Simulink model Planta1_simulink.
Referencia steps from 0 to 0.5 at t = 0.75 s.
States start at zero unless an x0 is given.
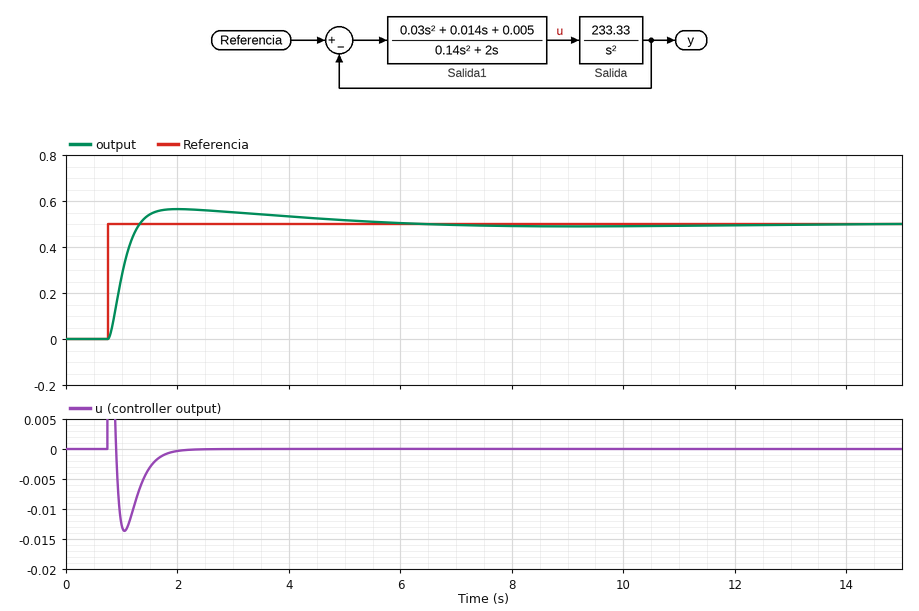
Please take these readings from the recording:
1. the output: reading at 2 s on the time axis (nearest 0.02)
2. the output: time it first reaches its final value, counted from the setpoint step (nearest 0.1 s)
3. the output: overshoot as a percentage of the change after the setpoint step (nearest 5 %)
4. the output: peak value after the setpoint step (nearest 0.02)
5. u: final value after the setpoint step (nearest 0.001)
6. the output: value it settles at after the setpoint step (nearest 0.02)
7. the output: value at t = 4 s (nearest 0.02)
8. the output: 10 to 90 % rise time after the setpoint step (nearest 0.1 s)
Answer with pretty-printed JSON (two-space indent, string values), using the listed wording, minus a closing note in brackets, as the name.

{
  "the output: reading at 2 s on the time axis": "0.56",
  "the output: time it first reaches its final value, counted from the setpoint step": "0.6 s",
  "the output: overshoot as a percentage of the change after the setpoint step": "15 %",
  "the output: peak value after the setpoint step": "0.56",
  "u: final value after the setpoint step": "0.000",
  "the output: value it settles at after the setpoint step": "0.50",
  "the output: value at t = 4 s": "0.54",
  "the output: 10 to 90 % rise time after the setpoint step": "0.4 s"
}
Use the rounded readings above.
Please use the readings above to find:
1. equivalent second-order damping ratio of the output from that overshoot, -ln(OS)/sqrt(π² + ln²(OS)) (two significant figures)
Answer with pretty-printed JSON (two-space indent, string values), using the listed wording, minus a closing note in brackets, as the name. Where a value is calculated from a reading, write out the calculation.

{
  "equivalent second-order damping ratio of the output from that overshoot, -ln(OS)/sqrt(π² + ln²(OS))": "ln(0.15) = -1.897; 1.897 / sqrt(9.870 + 3.599) = 0.52"
}
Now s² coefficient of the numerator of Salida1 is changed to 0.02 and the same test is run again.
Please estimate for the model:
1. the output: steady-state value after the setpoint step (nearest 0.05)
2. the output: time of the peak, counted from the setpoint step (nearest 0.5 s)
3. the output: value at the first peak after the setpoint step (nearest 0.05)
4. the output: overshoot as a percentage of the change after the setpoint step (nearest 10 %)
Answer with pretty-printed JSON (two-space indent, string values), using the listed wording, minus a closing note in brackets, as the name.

{
  "the output: steady-state value after the setpoint step": "0.50",
  "the output: time of the peak, counted from the setpoint step": "1.5 s",
  "the output: value at the first peak after the setpoint step": "0.60",
  "the output: overshoot as a percentage of the change after the setpoint step": "20 %"
}
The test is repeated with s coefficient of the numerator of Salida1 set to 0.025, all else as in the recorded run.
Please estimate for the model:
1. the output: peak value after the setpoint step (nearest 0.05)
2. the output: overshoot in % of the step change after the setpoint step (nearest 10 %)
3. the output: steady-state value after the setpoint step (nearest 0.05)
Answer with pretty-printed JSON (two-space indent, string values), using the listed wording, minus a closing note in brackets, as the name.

{
  "the output: peak value after the setpoint step": "0.60",
  "the output: overshoot in % of the step change after the setpoint step": "20 %",
  "the output: steady-state value after the setpoint step": "0.50"
}
